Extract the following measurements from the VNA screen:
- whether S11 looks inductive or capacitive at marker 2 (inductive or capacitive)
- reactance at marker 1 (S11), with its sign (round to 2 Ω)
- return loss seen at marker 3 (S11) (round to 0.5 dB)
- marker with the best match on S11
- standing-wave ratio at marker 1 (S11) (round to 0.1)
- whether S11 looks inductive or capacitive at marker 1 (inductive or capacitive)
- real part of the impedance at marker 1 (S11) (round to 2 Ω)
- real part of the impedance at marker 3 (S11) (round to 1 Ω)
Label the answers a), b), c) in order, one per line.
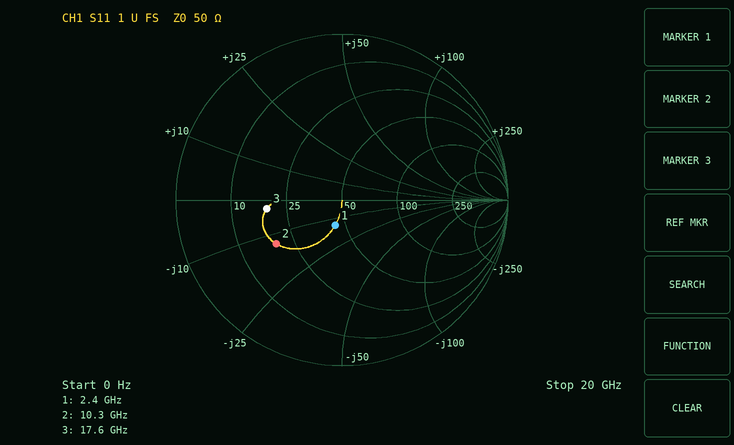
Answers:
a) capacitive
b) -14 Ω
c) 7.0 dB
d) marker 1
e) 1.4
f) capacitive
g) 44 Ω
h) 19 Ω
